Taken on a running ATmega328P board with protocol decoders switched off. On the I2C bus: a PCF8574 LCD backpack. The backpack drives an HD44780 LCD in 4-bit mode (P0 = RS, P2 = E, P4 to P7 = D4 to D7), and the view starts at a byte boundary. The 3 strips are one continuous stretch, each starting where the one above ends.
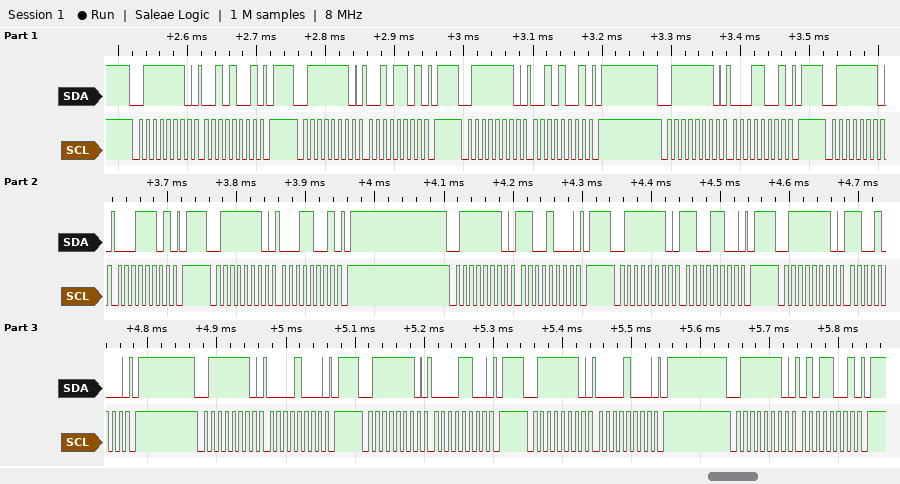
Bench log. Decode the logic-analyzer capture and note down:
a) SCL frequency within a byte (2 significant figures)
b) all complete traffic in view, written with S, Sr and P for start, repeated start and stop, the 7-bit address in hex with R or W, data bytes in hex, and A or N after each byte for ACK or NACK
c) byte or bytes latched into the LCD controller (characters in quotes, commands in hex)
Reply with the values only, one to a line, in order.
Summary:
100 kHz
S 3FW A 29 A P S 3FW A 2D A P S 3FW A 29 A P S 3FW A 19 A P S 3FW A 1D A P S 3FW A 19 A P S 3FW A C8 A P S 3FW A CC A P S 3FW A C8 A P S 3FW A 08 A P S 3FW A 0C A P S 3FW A 08 A P S 3FW A 59 A P
'!' 0xC0
